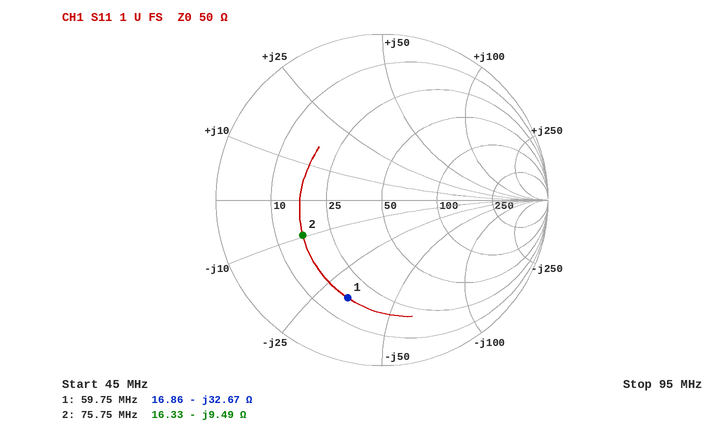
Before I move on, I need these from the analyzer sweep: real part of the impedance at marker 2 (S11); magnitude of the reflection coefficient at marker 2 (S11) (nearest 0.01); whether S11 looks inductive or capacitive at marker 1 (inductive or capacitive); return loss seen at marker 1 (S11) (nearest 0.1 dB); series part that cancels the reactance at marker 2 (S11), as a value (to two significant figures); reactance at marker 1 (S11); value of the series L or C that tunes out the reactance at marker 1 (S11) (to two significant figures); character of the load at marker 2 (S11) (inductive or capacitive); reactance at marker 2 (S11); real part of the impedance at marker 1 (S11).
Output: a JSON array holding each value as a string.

["16.33 Ω", "0.52", "capacitive", "4.1 dB", "20 nH", "-32.67 Ω", "87 nH", "capacitive", "-9.49 Ω", "16.86 Ω"]
